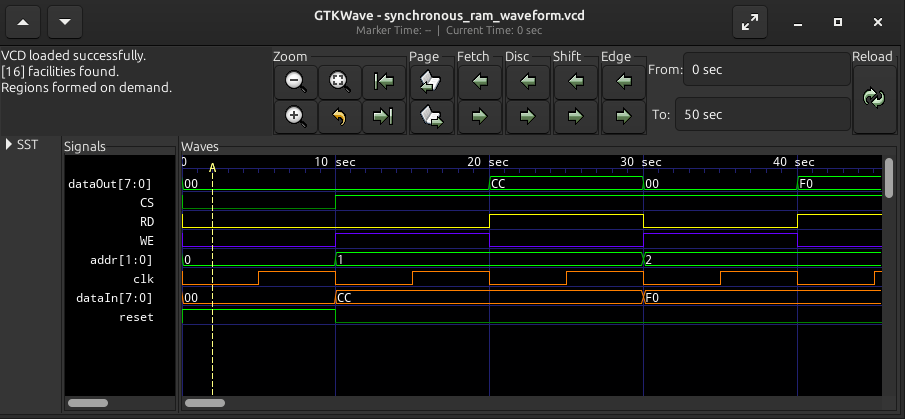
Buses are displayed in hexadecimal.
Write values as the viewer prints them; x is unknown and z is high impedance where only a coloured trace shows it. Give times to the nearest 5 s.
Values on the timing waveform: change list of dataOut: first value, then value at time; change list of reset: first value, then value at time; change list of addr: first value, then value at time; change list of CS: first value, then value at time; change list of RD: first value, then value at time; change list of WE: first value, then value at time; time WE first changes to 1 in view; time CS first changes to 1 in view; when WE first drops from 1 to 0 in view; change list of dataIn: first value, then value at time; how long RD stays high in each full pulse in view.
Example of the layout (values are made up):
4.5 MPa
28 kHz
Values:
00, CC at 20 s, 00 at 30 s, F0 at 40 s
1, 0 at 10 s
0, 1 at 10 s, 2 at 30 s
0, 1 at 10 s
0, 1 at 20 s, 0 at 30 s, 1 at 40 s
0, 1 at 10 s, 0 at 20 s, 1 at 30 s, 0 at 40 s
10 s
10 s
20 s
00, CC at 10 s, F0 at 30 s
10 s
